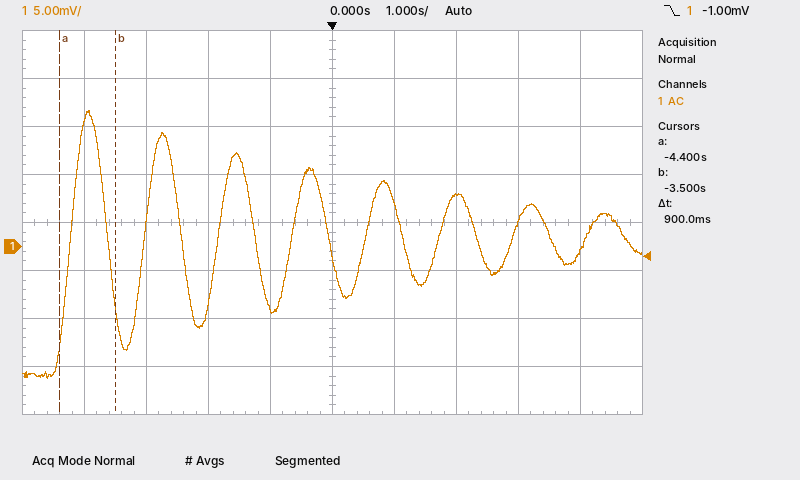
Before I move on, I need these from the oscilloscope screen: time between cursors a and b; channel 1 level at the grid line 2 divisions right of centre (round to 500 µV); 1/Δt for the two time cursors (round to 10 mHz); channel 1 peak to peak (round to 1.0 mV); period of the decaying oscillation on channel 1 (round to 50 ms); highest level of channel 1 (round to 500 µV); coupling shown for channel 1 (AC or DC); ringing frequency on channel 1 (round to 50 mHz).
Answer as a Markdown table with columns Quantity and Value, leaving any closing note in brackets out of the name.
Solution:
| Quantity | Value |
|---|---|
| time between cursors a and b | 900 ms |
| channel 1 level at the grid line 2 divisions right of centre | 5.5 mV |
| 1/Δt for the two time cursors | 1.11 Hz |
| channel 1 peak to peak | 28.0 mV |
| period of the decaying oscillation on channel 1 | 1.20 s |
| highest level of channel 1 | 14.0 mV |
| coupling shown for channel 1 | AC |
| ringing frequency on channel 1 | 850 mHz |
